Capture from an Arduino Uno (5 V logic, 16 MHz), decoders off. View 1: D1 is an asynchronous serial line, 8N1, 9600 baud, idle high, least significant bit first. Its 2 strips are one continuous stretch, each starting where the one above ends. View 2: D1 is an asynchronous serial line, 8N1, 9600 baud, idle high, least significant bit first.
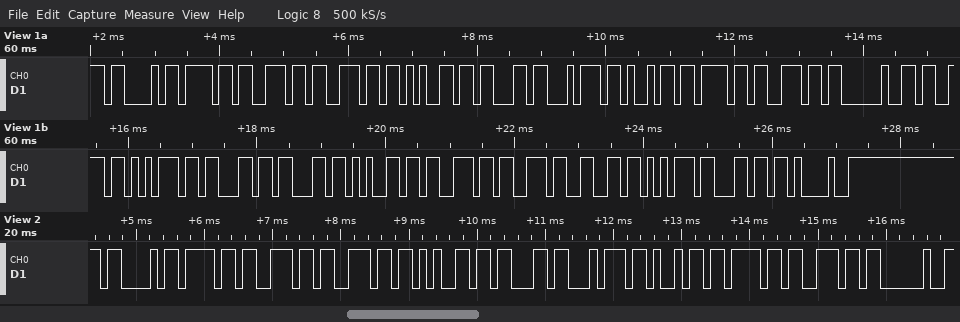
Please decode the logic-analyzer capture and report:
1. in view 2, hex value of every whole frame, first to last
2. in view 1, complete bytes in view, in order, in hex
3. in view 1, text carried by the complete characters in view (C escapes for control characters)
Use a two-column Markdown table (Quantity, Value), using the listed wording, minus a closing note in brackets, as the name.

| Quantity | Value |
|---|---|
| in view 2, hex value of every whole frame, first to last | 43 6F 6E 6E 65 63 74 69 6F 6E 20 |
| in view 1, complete bytes in view, in order, in hex | 0x43 0x6F 0x6E 0x6E 0x65 0x63 0x74 0x69 0x6F 0x6E 0x20 0x73 0x75 0x63 0x63 0x65 0x73 0x73 0x66 0x75 0x6C 0x21 |
| in view 1, text carried by the complete characters in view | "Connection successful!" |
